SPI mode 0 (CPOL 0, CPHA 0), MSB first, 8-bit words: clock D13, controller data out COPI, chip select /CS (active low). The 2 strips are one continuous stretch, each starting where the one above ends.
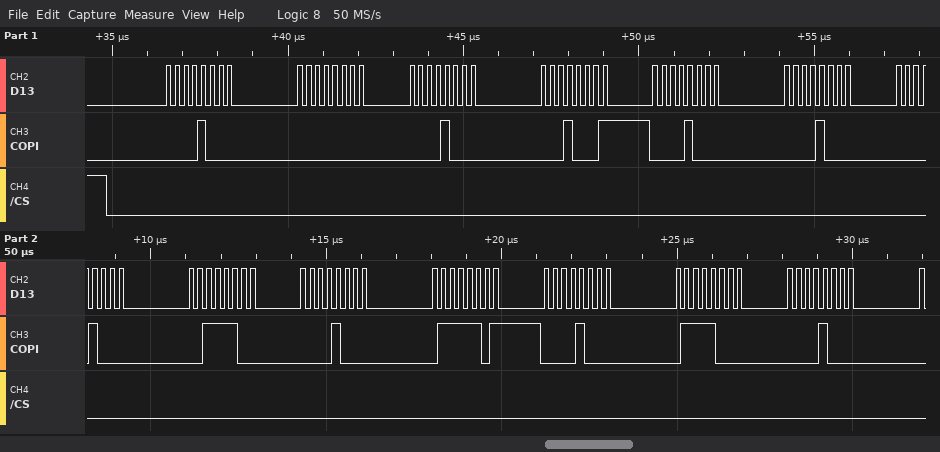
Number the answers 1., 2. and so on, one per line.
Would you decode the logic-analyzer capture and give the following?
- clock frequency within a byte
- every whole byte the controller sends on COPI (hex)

1. 4 MHz
2. 08 00 08 11 08 08 08 3C 08 7D 08 78 08
